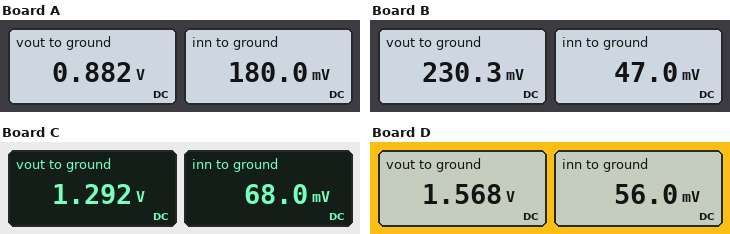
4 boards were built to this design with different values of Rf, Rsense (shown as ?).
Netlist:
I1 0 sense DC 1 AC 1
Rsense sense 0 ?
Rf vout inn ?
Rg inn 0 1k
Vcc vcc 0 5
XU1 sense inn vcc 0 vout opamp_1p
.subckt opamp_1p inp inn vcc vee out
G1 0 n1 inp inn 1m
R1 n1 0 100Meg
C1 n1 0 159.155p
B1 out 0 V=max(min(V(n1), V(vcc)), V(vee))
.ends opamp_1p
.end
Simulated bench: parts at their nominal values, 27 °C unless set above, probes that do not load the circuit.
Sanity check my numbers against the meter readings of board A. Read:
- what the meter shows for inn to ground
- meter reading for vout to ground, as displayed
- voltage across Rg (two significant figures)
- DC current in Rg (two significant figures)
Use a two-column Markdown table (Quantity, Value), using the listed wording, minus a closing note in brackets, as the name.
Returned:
| Quantity | Value |
|---|---|
| what the meter shows for inn to ground | 180.0 mV |
| meter reading for vout to ground, as displayed | 0.882 V |
| voltage across Rg | 180 mV |
| DC current in Rg | 180 µA |
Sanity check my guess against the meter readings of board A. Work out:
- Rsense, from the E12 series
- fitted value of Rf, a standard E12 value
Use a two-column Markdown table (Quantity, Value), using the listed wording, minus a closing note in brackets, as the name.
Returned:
| Quantity | Value |
|---|---|
| Rsense, from the E12 series | 0.18 Ω |
| fitted value of Rf, a standard E12 value | 3.9 kΩ |
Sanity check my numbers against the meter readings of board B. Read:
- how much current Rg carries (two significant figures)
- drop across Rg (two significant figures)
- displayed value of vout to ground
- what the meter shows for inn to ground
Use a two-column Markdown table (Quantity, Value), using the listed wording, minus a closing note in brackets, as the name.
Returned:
| Quantity | Value |
|---|---|
| how much current Rg carries | 47 µA |
| drop across Rg | 47 mV |
| displayed value of vout to ground | 230.3 mV |
| what the meter shows for inn to ground | 47.0 mV |
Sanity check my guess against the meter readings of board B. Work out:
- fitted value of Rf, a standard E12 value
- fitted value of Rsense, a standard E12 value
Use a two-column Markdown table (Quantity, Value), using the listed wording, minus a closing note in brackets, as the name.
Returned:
| Quantity | Value |
|---|---|
| fitted value of Rf, a standard E12 value | 3.9 kΩ |
| fitted value of Rsense, a standard E12 value | 0.047 Ω |
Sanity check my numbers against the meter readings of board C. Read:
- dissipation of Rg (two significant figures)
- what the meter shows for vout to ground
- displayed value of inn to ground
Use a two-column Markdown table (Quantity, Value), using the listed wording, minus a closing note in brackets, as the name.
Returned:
| Quantity | Value |
|---|---|
| dissipation of Rg | 4.6 µW |
| what the meter shows for vout to ground | 1.292 V |
| displayed value of inn to ground | 68.0 mV |
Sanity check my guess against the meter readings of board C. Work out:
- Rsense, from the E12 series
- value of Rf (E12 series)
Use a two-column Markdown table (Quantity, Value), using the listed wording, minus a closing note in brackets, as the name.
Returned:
| Quantity | Value |
|---|---|
| Rsense, from the E12 series | 0.068 Ω |
| value of Rf | 18 kΩ |
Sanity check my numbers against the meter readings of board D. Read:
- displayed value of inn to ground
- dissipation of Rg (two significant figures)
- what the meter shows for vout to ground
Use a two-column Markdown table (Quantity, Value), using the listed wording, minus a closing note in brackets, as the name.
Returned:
| Quantity | Value |
|---|---|
| displayed value of inn to ground | 56.0 mV |
| dissipation of Rg | 3.1 µW |
| what the meter shows for vout to ground | 1.568 V |
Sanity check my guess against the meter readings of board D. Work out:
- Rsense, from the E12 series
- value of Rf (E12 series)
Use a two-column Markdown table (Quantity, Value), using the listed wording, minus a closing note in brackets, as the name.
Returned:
| Quantity | Value |
|---|---|
| Rsense, from the E12 series | 0.056 Ω |
| value of Rf | 27 kΩ |
